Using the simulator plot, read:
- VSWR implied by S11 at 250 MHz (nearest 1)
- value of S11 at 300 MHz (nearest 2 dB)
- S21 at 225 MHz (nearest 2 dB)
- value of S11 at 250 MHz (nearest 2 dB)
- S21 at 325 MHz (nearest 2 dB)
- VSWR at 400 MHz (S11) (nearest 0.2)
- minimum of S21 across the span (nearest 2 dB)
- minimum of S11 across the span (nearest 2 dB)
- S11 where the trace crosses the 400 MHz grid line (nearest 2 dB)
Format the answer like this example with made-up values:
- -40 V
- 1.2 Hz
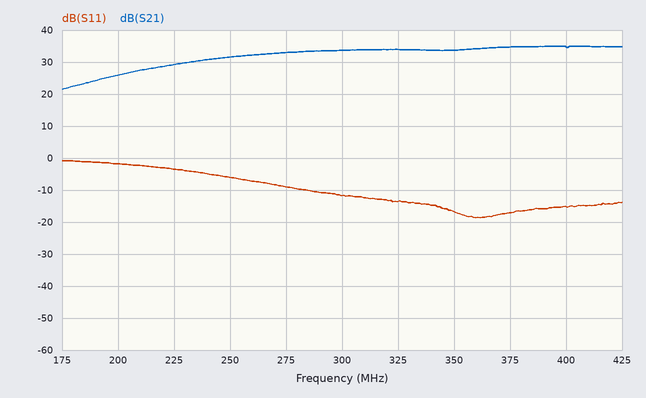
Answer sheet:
- 3
- -12 dB
- 30 dB
- -6 dB
- 34 dB
- 1.4
- 22 dB
- -18 dB
- -16 dB
